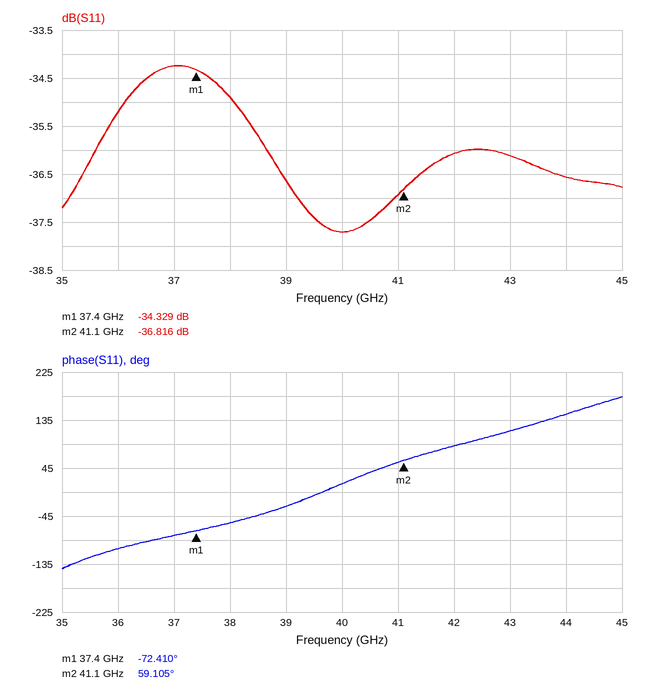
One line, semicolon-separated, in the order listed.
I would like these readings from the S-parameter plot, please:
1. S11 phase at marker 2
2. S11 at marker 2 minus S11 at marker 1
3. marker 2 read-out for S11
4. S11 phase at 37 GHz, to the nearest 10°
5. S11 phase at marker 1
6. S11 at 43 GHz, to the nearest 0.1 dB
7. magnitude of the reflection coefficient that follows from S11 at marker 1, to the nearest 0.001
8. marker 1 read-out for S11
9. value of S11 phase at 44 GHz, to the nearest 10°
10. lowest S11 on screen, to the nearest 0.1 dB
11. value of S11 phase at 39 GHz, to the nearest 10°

59.105°; -2.487 dB; -36.816 dB; -80°; -72.410°; -36.1 dB; 0.019; -34.329 dB; 150°; -37.7 dB; -30°
